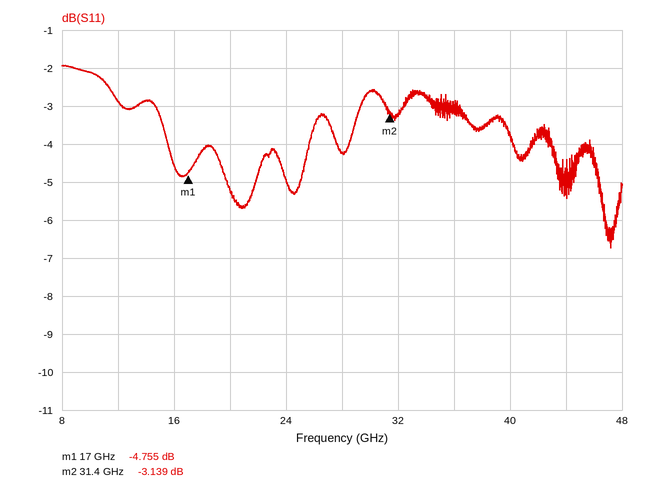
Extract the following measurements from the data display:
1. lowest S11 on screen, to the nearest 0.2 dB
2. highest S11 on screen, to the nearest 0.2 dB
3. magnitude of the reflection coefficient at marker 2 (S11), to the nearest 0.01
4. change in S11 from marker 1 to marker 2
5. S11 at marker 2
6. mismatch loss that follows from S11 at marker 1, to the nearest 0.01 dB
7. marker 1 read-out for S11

-6.8 dB
-2.0 dB
0.70
1.616 dB
-3.139 dB
1.77 dB
-4.755 dB
